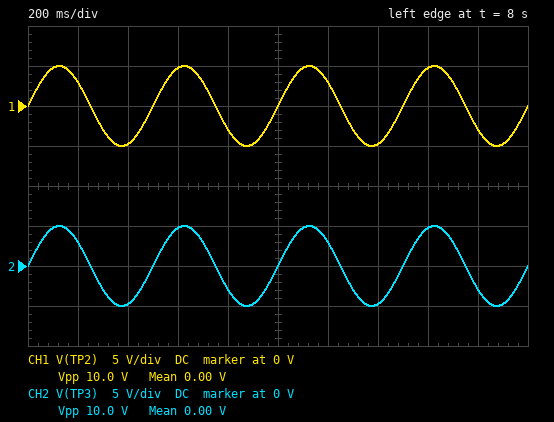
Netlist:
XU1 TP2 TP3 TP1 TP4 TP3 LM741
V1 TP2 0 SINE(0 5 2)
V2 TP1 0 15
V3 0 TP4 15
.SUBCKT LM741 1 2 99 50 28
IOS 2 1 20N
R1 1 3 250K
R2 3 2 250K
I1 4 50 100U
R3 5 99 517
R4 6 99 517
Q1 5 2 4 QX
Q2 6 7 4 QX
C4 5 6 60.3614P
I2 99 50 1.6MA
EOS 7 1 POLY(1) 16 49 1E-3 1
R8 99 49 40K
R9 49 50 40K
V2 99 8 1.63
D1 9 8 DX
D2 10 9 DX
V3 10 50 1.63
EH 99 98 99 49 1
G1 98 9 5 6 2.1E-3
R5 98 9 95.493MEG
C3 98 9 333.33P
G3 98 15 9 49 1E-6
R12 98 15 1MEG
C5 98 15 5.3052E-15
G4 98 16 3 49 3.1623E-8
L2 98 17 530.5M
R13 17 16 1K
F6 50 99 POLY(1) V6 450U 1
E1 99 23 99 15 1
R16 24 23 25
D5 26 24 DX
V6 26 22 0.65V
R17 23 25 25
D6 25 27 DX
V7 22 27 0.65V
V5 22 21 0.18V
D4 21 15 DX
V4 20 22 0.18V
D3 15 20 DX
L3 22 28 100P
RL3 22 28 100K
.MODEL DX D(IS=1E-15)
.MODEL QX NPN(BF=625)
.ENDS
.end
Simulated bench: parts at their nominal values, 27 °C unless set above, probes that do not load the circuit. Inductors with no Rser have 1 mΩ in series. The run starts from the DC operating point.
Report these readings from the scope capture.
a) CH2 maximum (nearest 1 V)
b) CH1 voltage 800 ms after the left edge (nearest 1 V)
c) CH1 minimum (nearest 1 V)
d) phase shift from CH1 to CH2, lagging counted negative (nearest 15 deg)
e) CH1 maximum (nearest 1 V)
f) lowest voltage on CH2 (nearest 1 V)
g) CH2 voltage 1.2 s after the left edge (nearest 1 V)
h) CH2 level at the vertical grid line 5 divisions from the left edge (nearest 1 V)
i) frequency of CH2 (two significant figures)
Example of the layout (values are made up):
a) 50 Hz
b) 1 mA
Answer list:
a) 5 V
b) -3 V
c) -5 V
d) 0 deg
e) 5 V
f) -5 V
g) 3 V
h) 0 V
i) 2.0 Hz
